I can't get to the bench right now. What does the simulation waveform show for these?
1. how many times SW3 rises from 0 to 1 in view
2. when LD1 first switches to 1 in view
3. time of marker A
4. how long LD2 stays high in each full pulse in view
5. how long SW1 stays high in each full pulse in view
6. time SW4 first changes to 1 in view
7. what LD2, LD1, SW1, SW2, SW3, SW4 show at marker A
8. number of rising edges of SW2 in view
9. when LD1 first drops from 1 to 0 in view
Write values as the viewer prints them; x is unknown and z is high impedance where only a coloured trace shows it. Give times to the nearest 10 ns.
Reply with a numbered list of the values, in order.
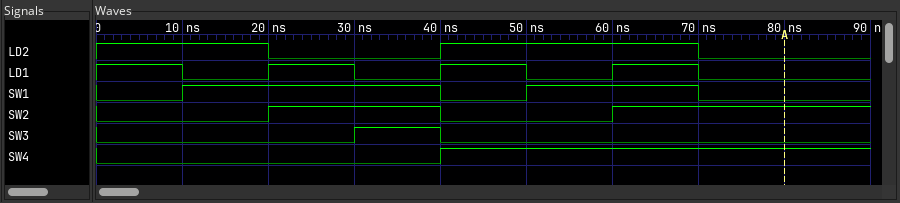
1. 1
2. 20 ns
3. 80 ns
4. 30 ns
5. 30 ns, 20 ns
6. 40 ns
7. LD2=0, LD1=0, SW1=0, SW2=1, SW3=0, SW4=1
8. 2
9. 10 ns
